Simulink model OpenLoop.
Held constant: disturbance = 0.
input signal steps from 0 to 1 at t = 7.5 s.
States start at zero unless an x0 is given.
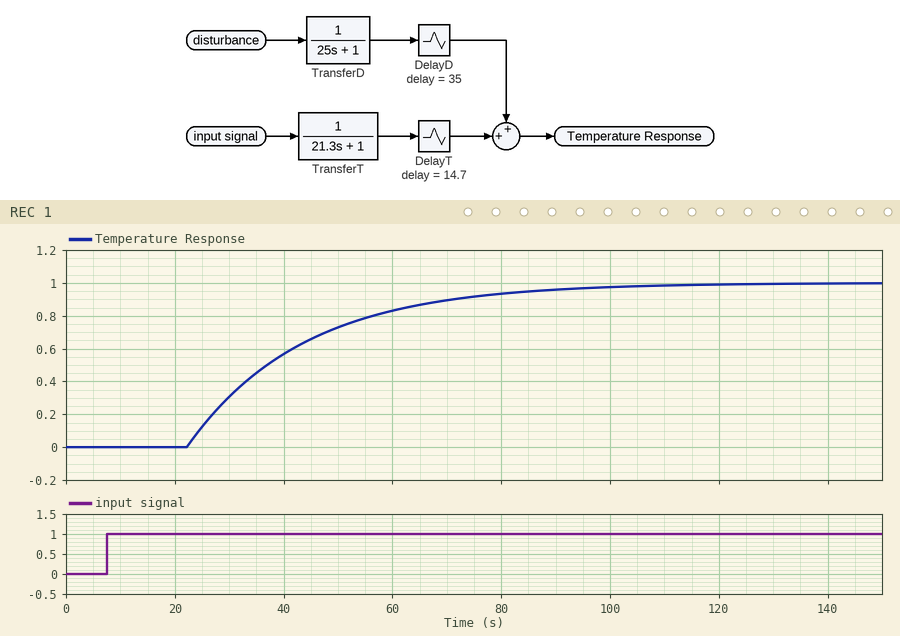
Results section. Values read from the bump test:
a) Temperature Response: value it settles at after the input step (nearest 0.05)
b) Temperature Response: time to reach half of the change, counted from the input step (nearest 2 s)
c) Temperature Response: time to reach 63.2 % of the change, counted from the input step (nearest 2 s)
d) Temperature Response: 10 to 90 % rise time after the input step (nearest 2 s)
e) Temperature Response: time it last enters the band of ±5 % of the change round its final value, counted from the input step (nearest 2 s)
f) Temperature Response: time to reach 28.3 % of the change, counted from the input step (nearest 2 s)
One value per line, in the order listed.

1.00
30 s
36 s
46 s
78 s
22 s
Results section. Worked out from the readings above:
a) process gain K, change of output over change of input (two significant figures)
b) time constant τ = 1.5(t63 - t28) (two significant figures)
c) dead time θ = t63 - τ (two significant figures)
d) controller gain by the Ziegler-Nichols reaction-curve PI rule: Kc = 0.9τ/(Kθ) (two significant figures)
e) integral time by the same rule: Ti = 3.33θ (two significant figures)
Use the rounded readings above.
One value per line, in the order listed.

1.0
21 s
15 s
1.3
50 s
